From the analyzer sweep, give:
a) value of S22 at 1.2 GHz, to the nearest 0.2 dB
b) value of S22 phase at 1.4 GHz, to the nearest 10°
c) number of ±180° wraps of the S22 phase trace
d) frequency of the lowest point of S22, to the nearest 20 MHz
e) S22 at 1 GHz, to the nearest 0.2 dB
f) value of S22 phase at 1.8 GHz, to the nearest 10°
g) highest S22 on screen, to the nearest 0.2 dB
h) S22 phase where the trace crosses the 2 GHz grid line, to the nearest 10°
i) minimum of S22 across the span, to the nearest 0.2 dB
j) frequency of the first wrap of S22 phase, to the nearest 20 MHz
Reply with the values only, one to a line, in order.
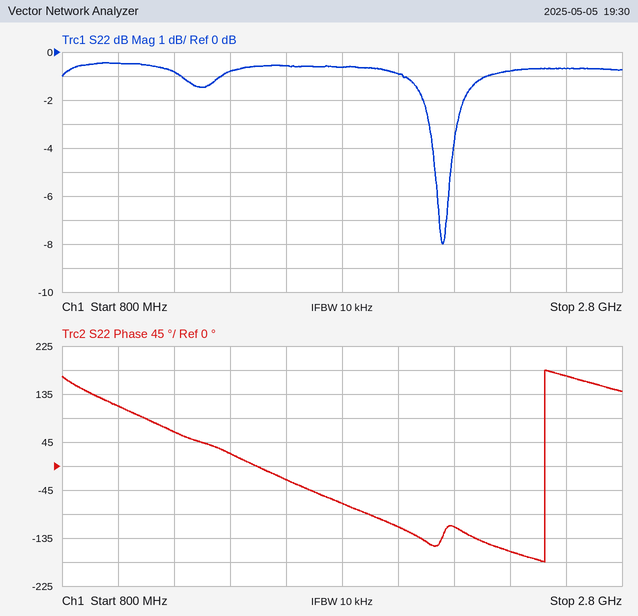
-0.8 dB
20°
1
2.16 GHz
-0.4 dB
-70°
-0.4 dB
-110°
-8.0 dB
2.52 GHz
